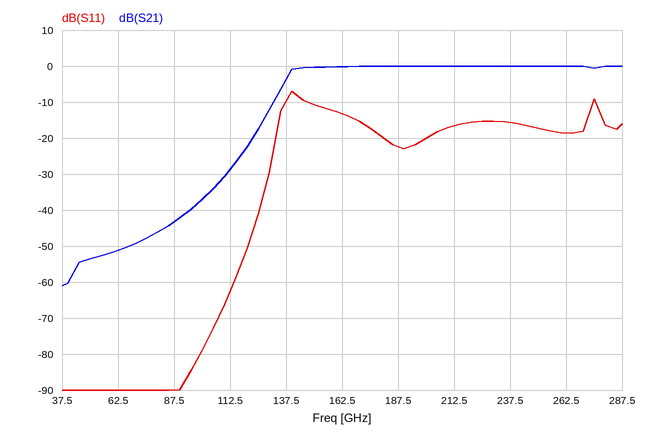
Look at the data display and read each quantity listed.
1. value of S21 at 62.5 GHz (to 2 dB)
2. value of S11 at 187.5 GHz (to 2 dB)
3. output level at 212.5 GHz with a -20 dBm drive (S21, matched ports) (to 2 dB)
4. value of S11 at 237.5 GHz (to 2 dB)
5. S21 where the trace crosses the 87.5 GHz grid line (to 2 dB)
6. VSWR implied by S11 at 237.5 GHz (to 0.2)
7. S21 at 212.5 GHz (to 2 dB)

-52 dB
-22 dB
-20 dBm
-16 dB
-44 dB
1.4
0 dB
